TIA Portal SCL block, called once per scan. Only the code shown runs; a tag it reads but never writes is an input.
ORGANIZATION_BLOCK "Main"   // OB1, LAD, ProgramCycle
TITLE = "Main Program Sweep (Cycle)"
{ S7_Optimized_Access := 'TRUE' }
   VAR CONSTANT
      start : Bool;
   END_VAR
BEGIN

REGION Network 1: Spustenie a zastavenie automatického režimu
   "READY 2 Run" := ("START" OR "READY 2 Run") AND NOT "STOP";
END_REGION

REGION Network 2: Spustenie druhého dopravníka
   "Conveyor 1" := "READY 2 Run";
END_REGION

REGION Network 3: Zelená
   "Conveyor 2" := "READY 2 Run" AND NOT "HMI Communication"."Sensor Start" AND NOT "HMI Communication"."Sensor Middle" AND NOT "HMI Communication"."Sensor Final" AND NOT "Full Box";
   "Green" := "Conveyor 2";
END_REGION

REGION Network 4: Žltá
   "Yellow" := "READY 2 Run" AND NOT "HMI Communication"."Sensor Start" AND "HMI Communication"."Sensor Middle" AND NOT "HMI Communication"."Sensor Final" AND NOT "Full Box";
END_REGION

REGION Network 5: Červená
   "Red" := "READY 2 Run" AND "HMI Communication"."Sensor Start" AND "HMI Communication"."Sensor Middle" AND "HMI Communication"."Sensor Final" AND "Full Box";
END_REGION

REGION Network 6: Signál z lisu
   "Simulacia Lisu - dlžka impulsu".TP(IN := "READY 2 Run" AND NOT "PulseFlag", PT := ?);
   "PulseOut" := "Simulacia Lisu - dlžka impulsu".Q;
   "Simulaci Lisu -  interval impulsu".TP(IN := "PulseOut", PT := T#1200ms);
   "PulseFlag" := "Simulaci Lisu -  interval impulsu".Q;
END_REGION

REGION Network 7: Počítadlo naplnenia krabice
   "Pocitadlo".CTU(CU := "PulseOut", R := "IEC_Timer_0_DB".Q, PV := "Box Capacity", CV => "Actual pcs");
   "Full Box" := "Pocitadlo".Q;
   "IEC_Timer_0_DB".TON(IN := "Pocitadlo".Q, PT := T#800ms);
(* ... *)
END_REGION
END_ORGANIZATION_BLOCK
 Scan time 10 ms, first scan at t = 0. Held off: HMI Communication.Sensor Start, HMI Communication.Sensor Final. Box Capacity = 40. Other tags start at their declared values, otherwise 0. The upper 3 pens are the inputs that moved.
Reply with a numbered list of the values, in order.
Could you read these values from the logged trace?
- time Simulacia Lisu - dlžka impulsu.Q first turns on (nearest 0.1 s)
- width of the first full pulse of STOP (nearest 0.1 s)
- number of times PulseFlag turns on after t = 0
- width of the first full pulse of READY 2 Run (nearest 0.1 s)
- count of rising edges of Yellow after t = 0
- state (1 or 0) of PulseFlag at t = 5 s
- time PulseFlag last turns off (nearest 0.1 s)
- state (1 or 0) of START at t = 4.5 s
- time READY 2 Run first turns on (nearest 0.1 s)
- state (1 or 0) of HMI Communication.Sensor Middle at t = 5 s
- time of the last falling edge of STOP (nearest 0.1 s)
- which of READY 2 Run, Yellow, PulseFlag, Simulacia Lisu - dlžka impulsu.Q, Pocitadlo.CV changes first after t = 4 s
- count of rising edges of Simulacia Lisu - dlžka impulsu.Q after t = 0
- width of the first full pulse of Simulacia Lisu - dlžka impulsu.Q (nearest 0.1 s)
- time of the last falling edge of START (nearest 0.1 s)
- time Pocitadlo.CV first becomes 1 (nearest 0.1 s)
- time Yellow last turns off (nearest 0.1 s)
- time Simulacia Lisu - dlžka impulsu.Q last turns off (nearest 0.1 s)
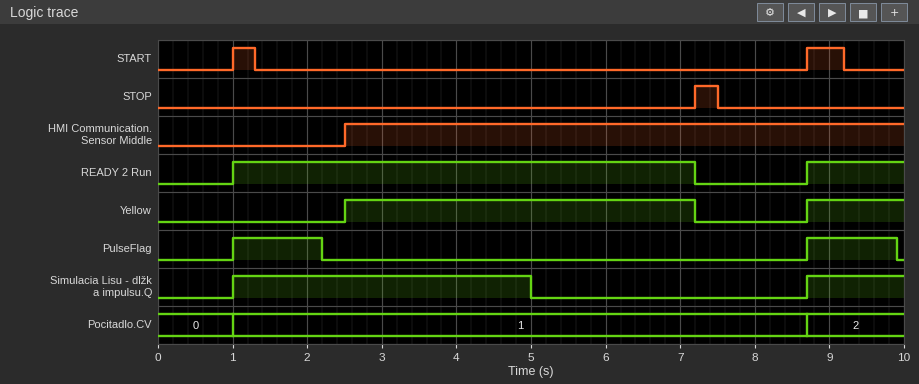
1. 1.0 s
2. 0.3 s
3. 2
4. 6.2 s
5. 2
6. 0
7. 9.9 s
8. 0
9. 1.0 s
10. 1
11. 7.5 s
12. Simulacia Lisu - dlžka impulsu.Q
13. 2
14. 4.0 s
15. 9.2 s
16. 1.0 s
17. 7.2 s
18. 5.0 s
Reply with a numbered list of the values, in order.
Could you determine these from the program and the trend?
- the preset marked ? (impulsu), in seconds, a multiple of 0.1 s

1. 4.0 s
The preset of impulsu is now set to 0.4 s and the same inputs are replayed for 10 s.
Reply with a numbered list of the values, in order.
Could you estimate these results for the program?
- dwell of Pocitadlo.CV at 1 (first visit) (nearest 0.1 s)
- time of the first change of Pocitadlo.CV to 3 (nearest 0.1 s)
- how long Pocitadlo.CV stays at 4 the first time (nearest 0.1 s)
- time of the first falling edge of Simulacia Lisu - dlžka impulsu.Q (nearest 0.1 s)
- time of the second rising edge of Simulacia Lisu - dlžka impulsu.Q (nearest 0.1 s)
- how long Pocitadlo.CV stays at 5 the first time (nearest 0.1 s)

1. 1.2 s
2. 3.4 s
3. 1.2 s
4. 1.4 s
5. 2.2 s
6. 1.2 s
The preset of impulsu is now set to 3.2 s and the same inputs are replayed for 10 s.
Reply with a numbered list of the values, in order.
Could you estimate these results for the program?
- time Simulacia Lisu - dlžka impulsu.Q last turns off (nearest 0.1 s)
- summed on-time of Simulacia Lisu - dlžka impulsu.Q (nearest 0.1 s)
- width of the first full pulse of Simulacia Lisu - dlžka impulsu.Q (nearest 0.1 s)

1. 4.2 s
2. 4.5 s
3. 3.2 s
